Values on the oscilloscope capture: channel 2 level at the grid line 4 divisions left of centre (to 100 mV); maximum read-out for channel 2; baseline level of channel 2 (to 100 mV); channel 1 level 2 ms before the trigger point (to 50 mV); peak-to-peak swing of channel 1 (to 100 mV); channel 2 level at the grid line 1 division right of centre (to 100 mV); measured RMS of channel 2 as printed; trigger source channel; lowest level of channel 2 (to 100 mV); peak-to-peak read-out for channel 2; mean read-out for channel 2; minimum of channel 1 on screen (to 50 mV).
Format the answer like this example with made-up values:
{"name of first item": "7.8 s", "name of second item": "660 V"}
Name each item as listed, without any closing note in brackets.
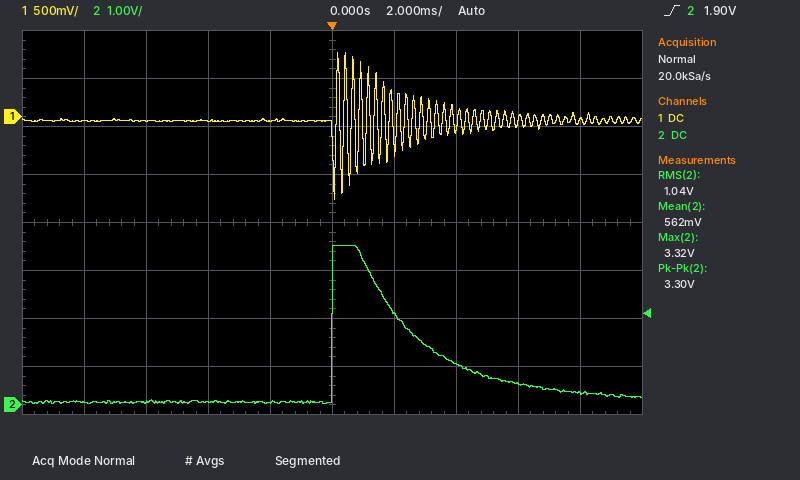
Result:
{"channel 2 level at the grid line 4 divisions left of centre": "100 mV", "maximum read-out for channel 2": "3.32 V", "baseline level of channel 2": "100 mV", "channel 1 level 2 ms before the trigger point": "-50 mV", "peak-to-peak swing of channel 1": "1.50 V", "channel 2 level at the grid line 1 division right of centre": "1.9 V", "measured RMS of channel 2 as printed": "1.04 V", "trigger source channel": "channel 2", "lowest level of channel 2": "0.0 V", "peak-to-peak read-out for channel 2": "3.30 V", "mean read-out for channel 2": "562 mV", "minimum of channel 1 on screen": "-850 mV"}
